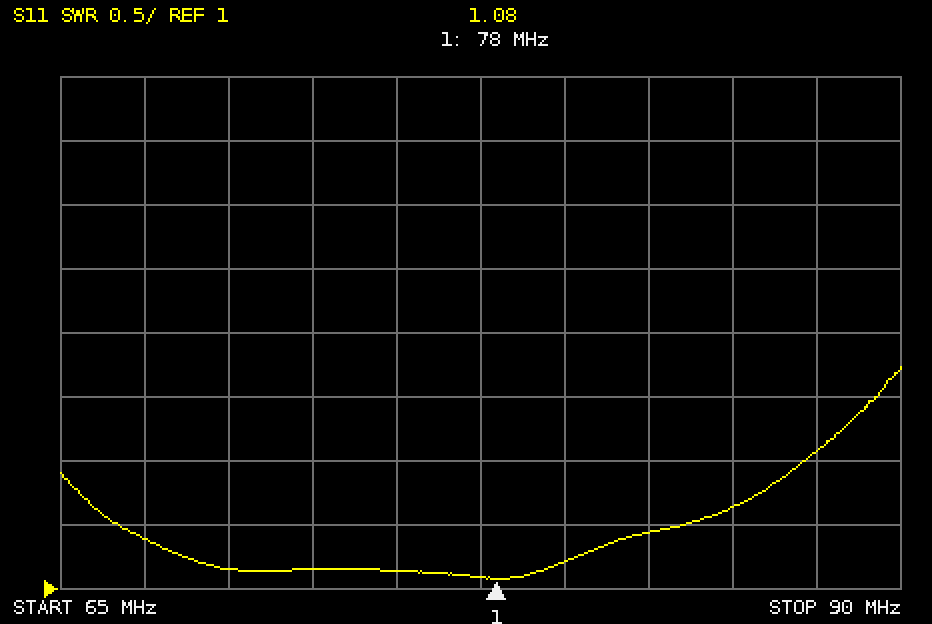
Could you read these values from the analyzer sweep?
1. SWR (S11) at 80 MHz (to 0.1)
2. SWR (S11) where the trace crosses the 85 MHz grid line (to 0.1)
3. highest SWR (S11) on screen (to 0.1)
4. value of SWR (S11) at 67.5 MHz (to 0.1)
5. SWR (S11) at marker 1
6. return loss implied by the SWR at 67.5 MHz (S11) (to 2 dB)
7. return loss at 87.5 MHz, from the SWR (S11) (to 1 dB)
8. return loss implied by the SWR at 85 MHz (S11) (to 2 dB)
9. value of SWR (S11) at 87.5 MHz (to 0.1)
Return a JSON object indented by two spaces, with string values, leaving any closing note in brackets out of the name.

{
  "SWR (S11) at 80 MHz": "1.2",
  "SWR (S11) where the trace crosses the 85 MHz grid line": "1.6",
  "highest SWR (S11) on screen": "2.7",
  "value of SWR (S11) at 67.5 MHz": "1.4",
  "SWR (S11) at marker 1": "1.08",
  "return loss implied by the SWR at 67.5 MHz (S11)": "16 dB",
  "return loss at 87.5 MHz, from the SWR (S11)": "9 dB",
  "return loss implied by the SWR at 85 MHz (S11)": "12 dB",
  "value of SWR (S11) at 87.5 MHz": "2.1"
}
